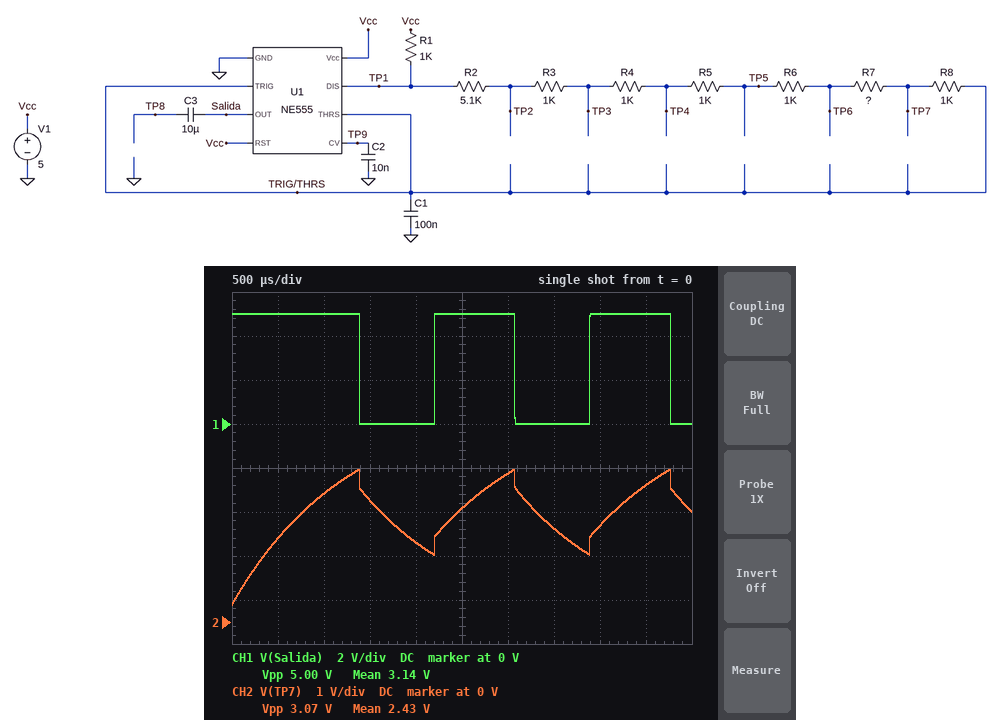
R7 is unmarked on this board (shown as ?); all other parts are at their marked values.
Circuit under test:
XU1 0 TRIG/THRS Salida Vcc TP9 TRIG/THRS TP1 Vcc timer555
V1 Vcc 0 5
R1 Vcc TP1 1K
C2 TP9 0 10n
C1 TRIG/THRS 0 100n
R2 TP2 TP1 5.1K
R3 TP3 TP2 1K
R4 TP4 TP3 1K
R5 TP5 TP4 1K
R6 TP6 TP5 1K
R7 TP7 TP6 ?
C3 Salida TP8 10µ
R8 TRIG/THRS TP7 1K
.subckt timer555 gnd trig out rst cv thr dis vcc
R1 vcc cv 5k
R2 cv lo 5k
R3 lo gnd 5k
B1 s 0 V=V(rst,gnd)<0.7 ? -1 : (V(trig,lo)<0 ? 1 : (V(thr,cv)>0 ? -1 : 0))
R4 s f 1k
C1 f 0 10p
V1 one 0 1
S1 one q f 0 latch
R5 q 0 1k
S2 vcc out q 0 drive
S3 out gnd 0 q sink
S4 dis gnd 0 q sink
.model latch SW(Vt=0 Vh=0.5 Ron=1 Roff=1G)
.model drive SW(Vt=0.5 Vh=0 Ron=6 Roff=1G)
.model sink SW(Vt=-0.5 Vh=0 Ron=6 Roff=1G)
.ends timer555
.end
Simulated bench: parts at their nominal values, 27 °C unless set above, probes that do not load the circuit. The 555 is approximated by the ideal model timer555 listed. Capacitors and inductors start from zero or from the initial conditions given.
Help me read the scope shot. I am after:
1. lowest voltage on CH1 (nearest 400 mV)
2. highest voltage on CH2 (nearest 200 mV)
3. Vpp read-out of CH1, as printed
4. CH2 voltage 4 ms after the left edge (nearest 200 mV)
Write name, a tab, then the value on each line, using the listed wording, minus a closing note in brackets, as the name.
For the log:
lowest voltage on CH1	0 V
highest voltage on CH2	3.4 V
Vpp read-out of CH1, as printed	5.00 V
CH2 voltage 4 ms after the left edge	2.2 V
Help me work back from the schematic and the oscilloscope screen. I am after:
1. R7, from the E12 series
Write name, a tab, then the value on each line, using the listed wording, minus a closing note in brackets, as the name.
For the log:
R7, from the E12 series	1.5 kΩ
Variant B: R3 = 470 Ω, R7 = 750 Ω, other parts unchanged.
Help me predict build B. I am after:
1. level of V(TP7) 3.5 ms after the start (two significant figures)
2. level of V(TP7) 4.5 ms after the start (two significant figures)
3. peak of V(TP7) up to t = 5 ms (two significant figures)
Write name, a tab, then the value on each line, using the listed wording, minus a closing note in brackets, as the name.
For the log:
level of V(TP7) 3.5 ms after the start	2.0 V
level of V(TP7) 4.5 ms after the start	2.4 V
peak of V(TP7) up to t = 5 ms	3.5 V
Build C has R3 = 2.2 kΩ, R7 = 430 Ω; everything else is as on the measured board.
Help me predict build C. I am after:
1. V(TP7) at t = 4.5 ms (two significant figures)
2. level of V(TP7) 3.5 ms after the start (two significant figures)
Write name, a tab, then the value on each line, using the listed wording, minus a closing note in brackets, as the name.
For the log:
V(TP7) at t = 4.5 ms	3.0 V
level of V(TP7) 3.5 ms after the start	2.2 V
